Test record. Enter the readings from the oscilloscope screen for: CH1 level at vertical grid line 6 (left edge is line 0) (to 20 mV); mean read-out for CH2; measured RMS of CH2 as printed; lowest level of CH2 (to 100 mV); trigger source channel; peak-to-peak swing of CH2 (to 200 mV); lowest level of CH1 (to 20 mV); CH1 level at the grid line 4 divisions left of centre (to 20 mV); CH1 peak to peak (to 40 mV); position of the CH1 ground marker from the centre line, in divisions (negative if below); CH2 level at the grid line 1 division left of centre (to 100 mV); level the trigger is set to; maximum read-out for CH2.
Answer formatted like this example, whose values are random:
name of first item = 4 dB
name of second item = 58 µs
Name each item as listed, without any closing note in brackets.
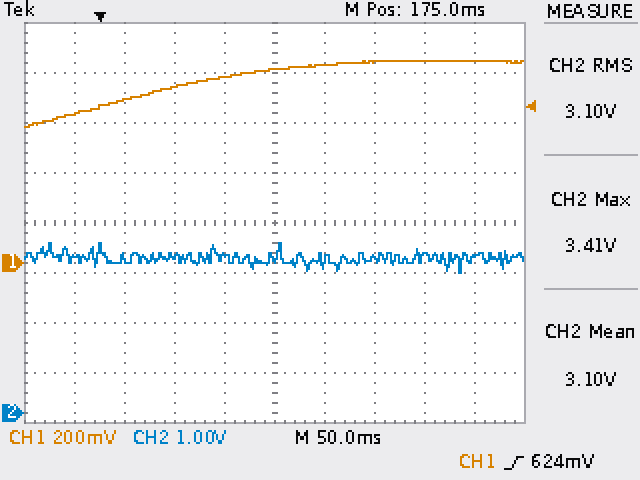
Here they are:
CH1 level at vertical grid line 6 (left edge is line 0) = 800 mV
mean read-out for CH2 = 3.10 V
measured RMS of CH2 as printed = 3.10 V
lowest level of CH2 = 2.8 V
trigger source channel = CH1
peak-to-peak swing of CH2 = 600 mV
lowest level of CH1 = 540 mV
CH1 level at the grid line 4 divisions left of centre = 600 mV
CH1 peak to peak = 280 mV
position of the CH1 ground marker from the centre line, in divisions = -0.8 div
CH2 level at the grid line 1 division left of centre = 3.1 V
level the trigger is set to = 624 mV
maximum read-out for CH2 = 3.41 V
